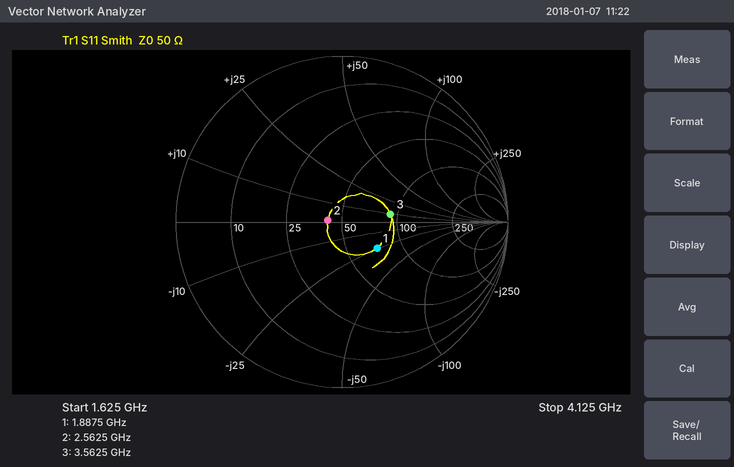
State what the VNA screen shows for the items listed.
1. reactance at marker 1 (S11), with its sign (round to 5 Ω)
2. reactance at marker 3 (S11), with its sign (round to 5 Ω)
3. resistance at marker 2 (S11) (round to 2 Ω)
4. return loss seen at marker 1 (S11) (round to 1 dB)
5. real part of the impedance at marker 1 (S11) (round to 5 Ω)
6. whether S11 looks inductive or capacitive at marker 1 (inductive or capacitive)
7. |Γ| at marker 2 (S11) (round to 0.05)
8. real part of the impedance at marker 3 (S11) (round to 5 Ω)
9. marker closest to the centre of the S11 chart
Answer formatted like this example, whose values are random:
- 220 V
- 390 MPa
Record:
- -25 Ω
- +10 Ω
- 42 Ω
- 12 dB
- 70 Ω
- capacitive
- 0.10
- 90 Ω
- marker 2
